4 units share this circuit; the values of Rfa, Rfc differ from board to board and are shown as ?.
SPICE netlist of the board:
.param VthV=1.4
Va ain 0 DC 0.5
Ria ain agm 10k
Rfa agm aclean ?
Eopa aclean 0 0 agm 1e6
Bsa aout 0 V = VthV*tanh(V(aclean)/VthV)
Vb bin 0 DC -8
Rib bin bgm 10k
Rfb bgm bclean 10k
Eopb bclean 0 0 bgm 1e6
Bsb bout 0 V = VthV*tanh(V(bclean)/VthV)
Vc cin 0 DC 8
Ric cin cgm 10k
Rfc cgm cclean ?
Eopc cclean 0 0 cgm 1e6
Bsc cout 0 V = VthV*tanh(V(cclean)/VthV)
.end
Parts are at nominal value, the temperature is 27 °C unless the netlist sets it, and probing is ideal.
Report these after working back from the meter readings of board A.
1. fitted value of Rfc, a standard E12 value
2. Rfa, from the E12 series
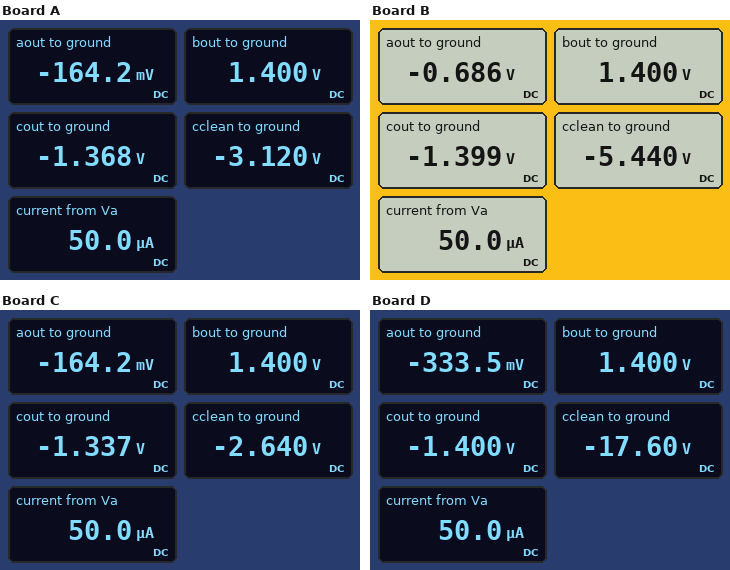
3.9 kΩ
3.3 kΩ
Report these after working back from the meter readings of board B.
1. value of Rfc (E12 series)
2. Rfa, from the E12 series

6.8 kΩ
15 kΩ
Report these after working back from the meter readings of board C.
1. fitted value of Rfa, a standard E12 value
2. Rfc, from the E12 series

3.3 kΩ
3.3 kΩ
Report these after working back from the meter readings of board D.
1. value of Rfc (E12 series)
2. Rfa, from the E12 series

22 kΩ
6.8 kΩ
